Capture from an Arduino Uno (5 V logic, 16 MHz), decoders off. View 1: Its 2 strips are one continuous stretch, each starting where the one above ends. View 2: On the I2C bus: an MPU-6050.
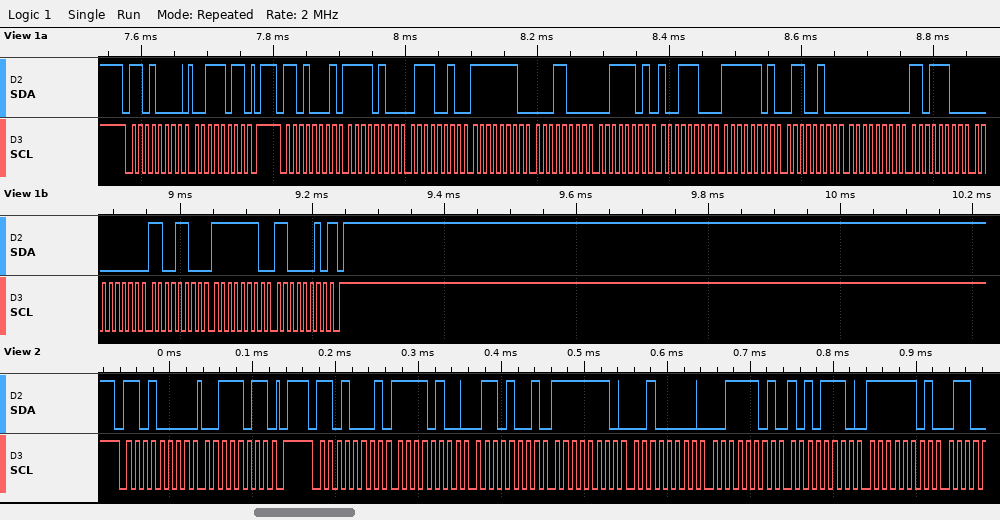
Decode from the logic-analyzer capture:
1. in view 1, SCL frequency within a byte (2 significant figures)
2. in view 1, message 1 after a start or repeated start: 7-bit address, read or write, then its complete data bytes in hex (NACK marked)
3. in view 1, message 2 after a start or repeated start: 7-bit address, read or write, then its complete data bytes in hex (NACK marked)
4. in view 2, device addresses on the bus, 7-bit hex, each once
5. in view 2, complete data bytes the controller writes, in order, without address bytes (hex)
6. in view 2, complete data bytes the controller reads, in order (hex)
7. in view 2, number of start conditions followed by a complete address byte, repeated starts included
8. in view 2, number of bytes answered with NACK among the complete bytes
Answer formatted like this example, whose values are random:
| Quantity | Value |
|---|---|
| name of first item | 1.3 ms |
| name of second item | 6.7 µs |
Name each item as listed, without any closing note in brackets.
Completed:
| Quantity | Value |
|---|---|
| in view 1, SCL frequency within a byte | 100 kHz |
| in view 1, message 1 after a start or repeated start: 7-bit address, read or write, then its complete data bytes in hex | 0x68 write: 3B |
| in view 1, message 2 after a start or repeated start: 7-bit address, read or write, then its complete data bytes in hex | 0x68 read: F4 72 FE 18 3D 9C FD 64 00 DC 00 CC FE C2 NACK |
| in view 2, device addresses on the bus, 7-bit hex, each once | 0x68 |
| in view 2, complete data bytes the controller writes, in order, without address bytes | 3B |
| in view 2, complete data bytes the controller reads, in order | F4 69 FE 20 3D AE FD |
| in view 2, number of start conditions followed by a complete address byte, repeated starts included | 2 |
| in view 2, number of bytes answered with NACK among the complete bytes | 0 |
